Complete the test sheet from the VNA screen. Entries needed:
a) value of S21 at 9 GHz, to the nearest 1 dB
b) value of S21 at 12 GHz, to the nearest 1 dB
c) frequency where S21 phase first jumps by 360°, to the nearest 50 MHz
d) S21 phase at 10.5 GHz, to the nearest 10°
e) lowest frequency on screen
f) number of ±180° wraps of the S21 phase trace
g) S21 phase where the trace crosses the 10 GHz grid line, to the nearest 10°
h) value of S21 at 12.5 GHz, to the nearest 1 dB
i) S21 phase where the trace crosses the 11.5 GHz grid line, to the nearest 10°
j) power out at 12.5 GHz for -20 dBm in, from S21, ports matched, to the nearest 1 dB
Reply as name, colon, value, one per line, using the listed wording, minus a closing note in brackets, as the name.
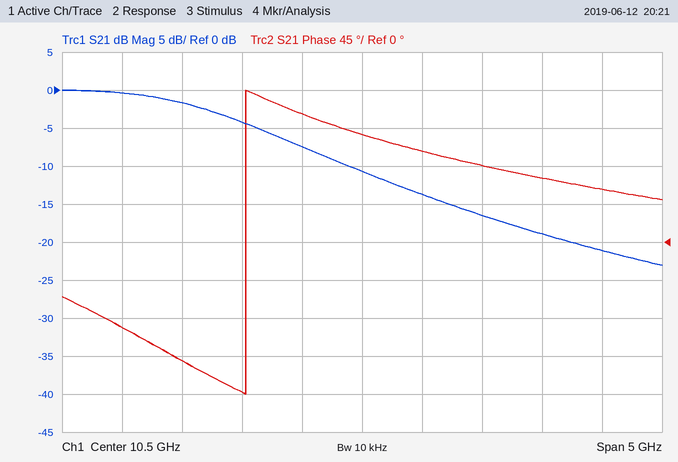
value of S21 at 9 GHz, to the nearest 1 dB: -2 dB
value of S21 at 12 GHz, to the nearest 1 dB: -19 dB
frequency where S21 phase first jumps by 360°, to the nearest 50 MHz: 9.55 GHz
S21 phase at 10.5 GHz, to the nearest 10°: 130°
lowest frequency on screen: 8 GHz
number of ±180° wraps of the S21 phase trace: 1
S21 phase where the trace crosses the 10 GHz grid line, to the nearest 10°: 150°
value of S21 at 12.5 GHz, to the nearest 1 dB: -21 dB
S21 phase where the trace crosses the 11.5 GHz grid line, to the nearest 10°: 90°
power out at 12.5 GHz for -20 dBm in, from S21, ports matched, to the nearest 1 dB: -41 dBm
